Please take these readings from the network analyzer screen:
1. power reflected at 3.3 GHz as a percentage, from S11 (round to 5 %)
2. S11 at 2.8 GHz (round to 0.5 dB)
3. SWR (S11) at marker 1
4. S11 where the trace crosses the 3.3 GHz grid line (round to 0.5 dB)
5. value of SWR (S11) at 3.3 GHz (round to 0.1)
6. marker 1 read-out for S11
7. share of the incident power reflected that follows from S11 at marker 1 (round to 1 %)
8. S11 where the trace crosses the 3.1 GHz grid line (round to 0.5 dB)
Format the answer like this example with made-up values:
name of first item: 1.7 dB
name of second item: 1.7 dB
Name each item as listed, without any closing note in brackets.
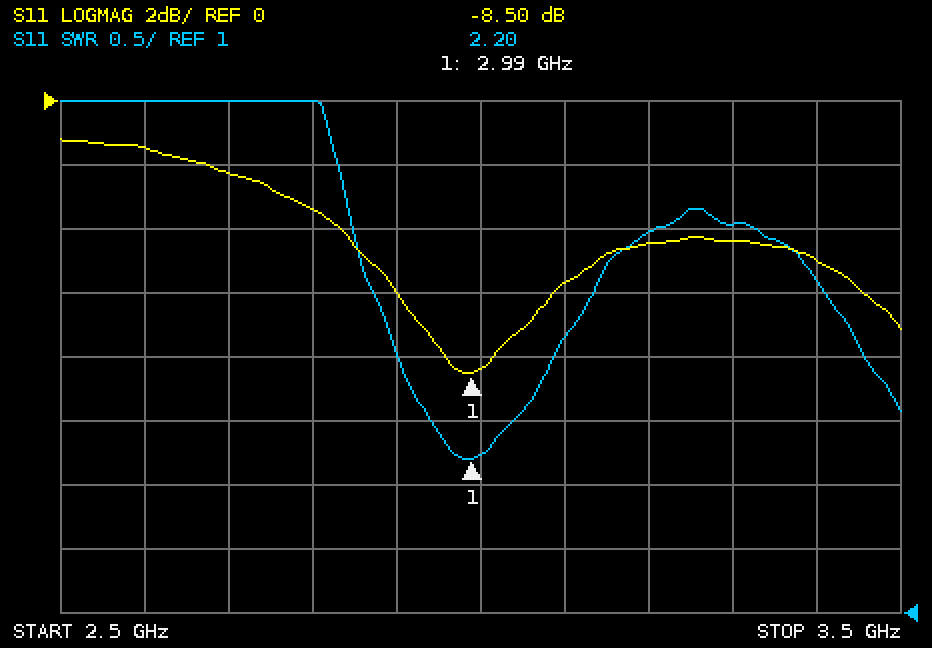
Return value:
power reflected at 3.3 GHz as a percentage, from S11: 35 %
S11 at 2.8 GHz: -3.5 dB
SWR (S11) at marker 1: 2.20
S11 where the trace crosses the 3.3 GHz grid line: -4.5 dB
value of SWR (S11) at 3.3 GHz: 4.0
marker 1 read-out for S11: -8.50 dB
share of the incident power reflected that follows from S11 at marker 1: 14 %
S11 where the trace crosses the 3.1 GHz grid line: -5.5 dB
